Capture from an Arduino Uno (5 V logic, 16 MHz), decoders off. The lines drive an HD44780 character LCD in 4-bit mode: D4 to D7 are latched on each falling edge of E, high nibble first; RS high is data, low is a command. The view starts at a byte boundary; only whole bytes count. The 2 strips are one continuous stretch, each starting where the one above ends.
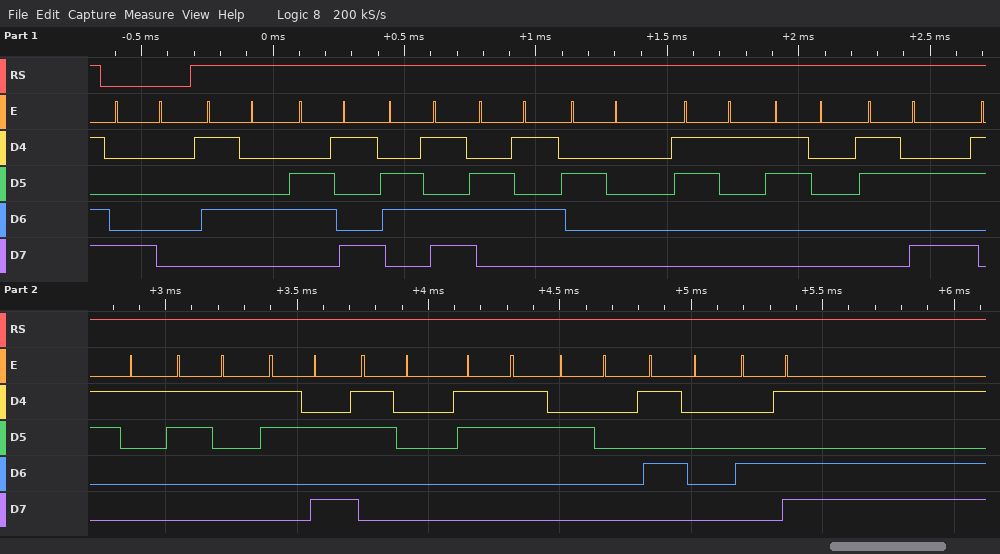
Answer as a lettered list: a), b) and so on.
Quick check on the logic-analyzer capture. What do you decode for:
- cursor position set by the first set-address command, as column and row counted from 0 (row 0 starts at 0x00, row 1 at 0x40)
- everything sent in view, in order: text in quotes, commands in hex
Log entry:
a) column 0, row 0
b) 0x80 "Time 10:11:03 PM"
